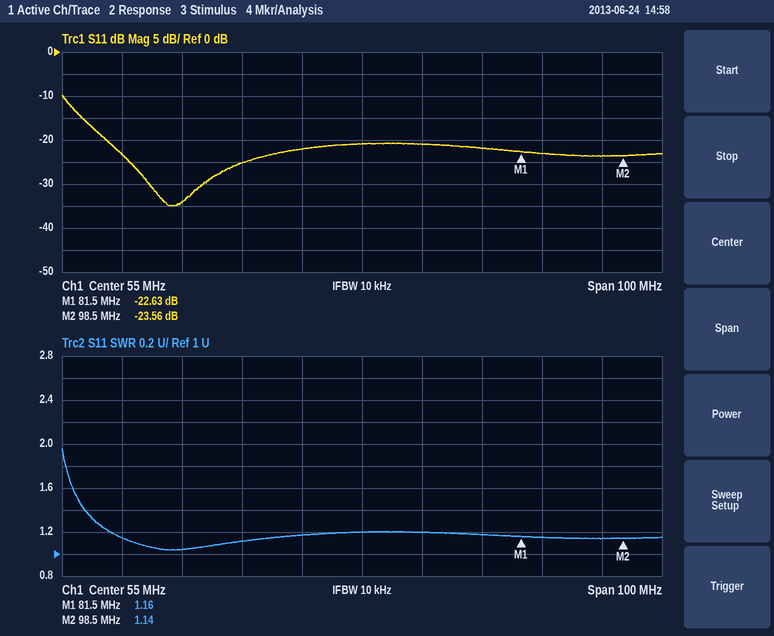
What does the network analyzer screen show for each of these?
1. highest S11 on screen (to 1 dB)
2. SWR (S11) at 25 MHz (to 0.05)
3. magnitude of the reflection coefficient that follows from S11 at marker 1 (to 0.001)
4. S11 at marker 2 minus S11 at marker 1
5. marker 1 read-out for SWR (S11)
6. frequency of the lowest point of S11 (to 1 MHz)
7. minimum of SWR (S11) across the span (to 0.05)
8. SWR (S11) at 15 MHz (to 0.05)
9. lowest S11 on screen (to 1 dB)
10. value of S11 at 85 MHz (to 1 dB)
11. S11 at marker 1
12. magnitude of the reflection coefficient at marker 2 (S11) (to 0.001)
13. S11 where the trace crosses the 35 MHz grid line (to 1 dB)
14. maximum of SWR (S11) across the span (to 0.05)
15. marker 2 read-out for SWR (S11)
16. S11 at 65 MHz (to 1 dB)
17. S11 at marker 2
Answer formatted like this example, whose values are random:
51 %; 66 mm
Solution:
-10 dB; 1.05; 0.074; -0.93 dB; 1.16; 23 MHz; 1.05; 1.15; -35 dB; -23 dB; -22.63 dB; 0.066; -25 dB; 1.95; 1.14; -21 dB; -23.56 dB
